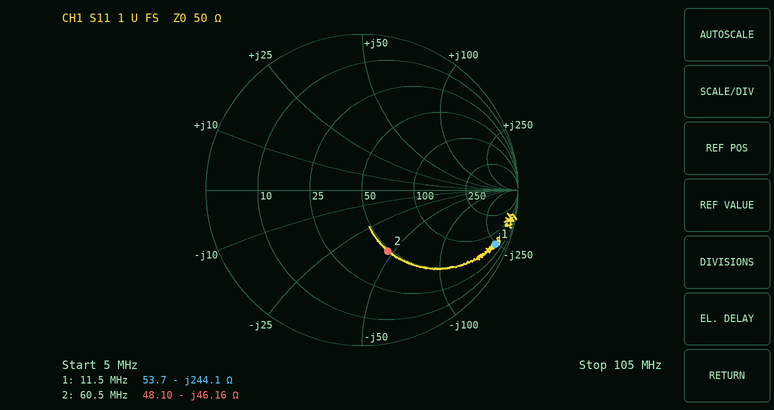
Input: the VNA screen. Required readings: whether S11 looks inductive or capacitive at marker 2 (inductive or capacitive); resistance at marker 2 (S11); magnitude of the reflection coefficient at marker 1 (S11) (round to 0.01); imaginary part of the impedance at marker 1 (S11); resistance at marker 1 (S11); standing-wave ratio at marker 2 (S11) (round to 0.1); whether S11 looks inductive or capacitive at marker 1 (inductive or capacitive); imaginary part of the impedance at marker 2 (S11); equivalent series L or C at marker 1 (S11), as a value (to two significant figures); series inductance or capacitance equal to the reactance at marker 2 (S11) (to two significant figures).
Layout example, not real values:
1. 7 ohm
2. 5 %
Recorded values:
1. capacitive
2. 48.10 Ω
3. 0.92
4. -244.1 Ω
5. 53.7 Ω
6. 2.5
7. capacitive
8. -46.16 Ω
9. 57 pF
10. 57 pF
